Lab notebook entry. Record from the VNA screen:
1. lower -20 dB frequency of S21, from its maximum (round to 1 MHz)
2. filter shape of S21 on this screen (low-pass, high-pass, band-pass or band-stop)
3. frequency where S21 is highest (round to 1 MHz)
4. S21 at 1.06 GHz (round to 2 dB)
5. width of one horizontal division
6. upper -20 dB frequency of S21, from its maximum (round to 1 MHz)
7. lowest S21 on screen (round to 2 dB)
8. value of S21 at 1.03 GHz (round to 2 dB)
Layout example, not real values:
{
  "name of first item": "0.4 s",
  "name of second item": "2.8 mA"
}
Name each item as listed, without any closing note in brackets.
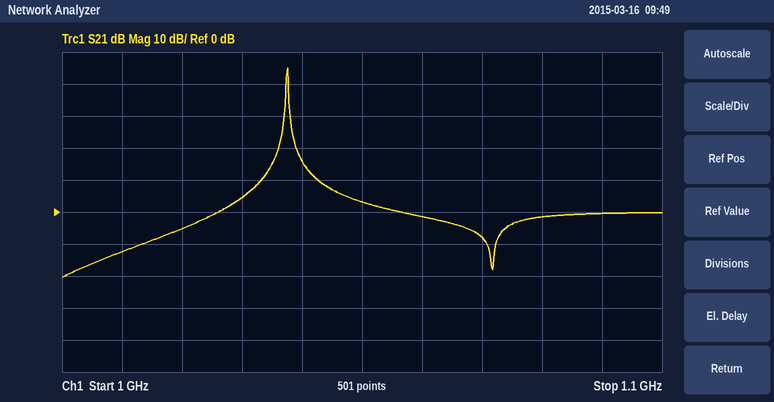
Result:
{
  "lower -20 dB frequency of S21, from its maximum": "1.037 GHz",
  "filter shape of S21 on this screen": "band-pass",
  "frequency where S21 is highest": "1.038 GHz",
  "S21 at 1.06 GHz": "-2 dB",
  "width of one horizontal division": "10 MHz",
  "upper -20 dB frequency of S21, from its maximum": "1.038 GHz",
  "lowest S21 on screen": "-20 dB",
  "value of S21 at 1.03 GHz": "4 dB"
}
